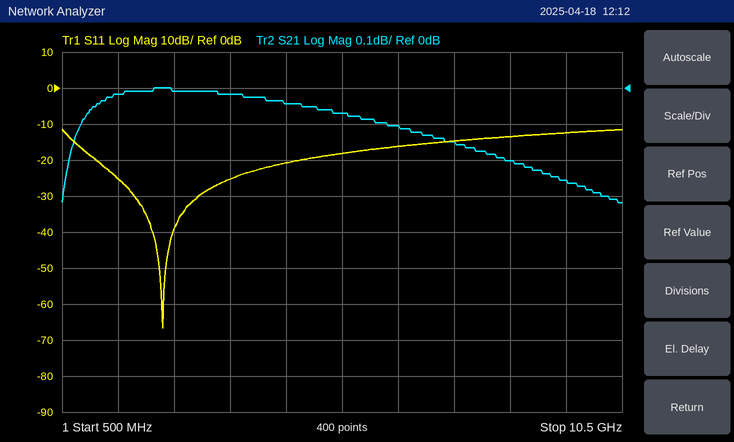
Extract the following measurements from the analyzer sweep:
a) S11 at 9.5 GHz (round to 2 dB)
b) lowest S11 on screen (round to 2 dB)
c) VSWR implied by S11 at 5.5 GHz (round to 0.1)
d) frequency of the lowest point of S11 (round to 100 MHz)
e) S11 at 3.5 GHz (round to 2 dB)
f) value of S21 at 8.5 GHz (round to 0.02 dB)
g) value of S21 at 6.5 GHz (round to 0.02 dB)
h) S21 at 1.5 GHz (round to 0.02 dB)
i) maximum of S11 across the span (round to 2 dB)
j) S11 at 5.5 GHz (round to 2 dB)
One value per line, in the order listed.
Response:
-12 dB
-66 dB
1.3
2.3 GHz
-26 dB
-0.20 dB
-0.10 dB
-0.02 dB
-12 dB
-18 dB
